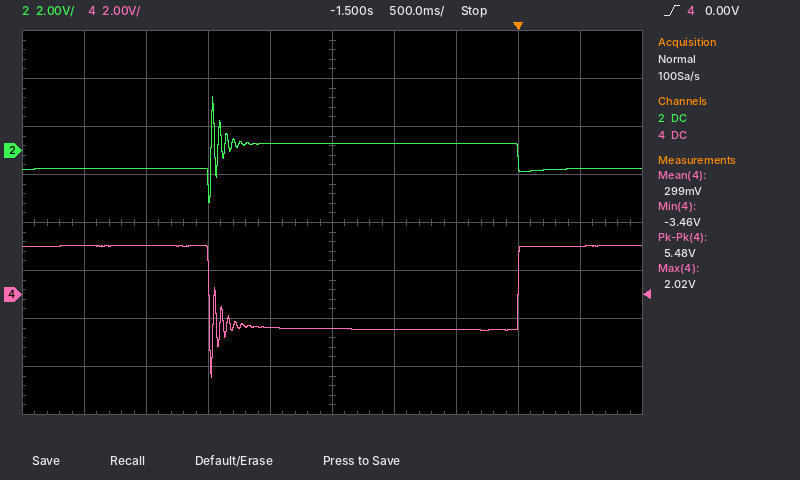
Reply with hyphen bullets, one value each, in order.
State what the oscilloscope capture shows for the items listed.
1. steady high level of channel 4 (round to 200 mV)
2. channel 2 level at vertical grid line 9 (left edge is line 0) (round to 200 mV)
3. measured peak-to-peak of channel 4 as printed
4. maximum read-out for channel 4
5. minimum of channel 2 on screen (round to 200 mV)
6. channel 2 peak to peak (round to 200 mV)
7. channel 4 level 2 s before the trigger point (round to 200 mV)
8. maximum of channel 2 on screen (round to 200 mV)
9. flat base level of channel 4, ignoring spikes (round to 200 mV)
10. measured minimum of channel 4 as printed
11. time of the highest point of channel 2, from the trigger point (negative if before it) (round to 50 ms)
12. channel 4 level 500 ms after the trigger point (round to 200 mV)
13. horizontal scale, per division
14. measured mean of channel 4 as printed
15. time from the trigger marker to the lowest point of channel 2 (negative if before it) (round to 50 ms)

- 2.0 V
- -800 mV
- 5.48 V
- 2.02 V
- -2.2 V
- 4.4 V
- -1.4 V
- 2.2 V
- -1.4 V
- -3.46 V
- -2.45 s
- 2.0 V
- 500 ms
- 299 mV
- -2.50 s
